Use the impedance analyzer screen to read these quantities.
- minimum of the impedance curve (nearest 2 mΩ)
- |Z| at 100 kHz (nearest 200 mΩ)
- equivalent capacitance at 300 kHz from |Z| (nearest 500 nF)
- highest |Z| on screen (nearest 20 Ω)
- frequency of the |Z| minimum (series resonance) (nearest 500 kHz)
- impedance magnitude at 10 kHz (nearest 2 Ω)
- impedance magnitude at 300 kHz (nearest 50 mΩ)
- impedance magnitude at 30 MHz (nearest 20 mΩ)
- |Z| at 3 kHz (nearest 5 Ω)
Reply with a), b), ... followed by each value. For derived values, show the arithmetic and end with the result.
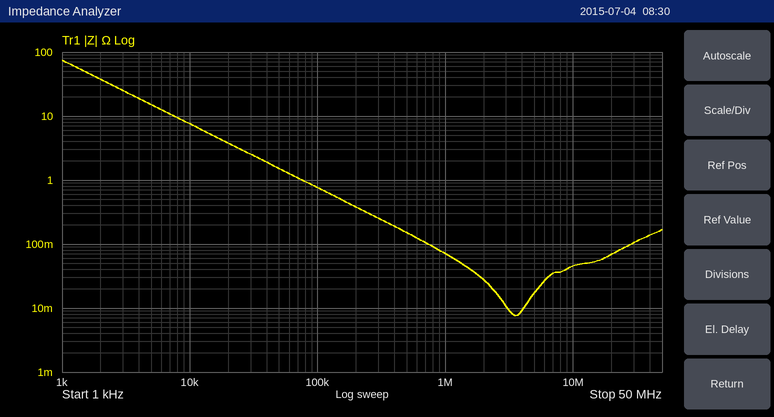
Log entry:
a) 8 mΩ
b) 800 mΩ
c) C = 1/(2π × 300 kHz × 250 mΩ) ≈ 2.12 µF, so 2.0 µF to the nearest 500 nF
d) 80 Ω
e) 3.5 MHz
f) 8 Ω
g) 250 mΩ
h) 100 mΩ
i) 25 Ω
